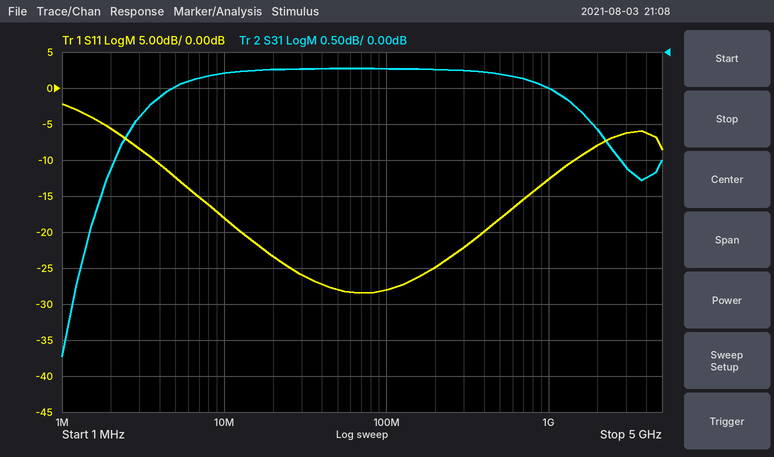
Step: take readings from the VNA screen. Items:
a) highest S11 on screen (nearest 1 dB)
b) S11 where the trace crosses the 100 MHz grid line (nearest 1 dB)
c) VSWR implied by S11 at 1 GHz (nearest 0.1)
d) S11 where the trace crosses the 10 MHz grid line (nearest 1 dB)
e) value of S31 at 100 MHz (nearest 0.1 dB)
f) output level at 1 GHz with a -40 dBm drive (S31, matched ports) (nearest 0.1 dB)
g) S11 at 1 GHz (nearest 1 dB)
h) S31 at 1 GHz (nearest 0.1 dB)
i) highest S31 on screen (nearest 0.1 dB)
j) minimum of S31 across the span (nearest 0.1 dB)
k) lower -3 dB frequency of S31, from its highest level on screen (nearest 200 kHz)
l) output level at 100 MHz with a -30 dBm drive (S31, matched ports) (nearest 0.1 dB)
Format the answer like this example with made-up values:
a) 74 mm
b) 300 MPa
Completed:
a) -2 dB
b) -28 dB
c) 1.6
d) -18 dB
e) -0.2 dB
f) -40.5 dBm
g) -13 dB
h) -0.5 dB
i) -0.2 dB
j) -4.2 dB
k) 1.2 MHz
l) -30.2 dBm
